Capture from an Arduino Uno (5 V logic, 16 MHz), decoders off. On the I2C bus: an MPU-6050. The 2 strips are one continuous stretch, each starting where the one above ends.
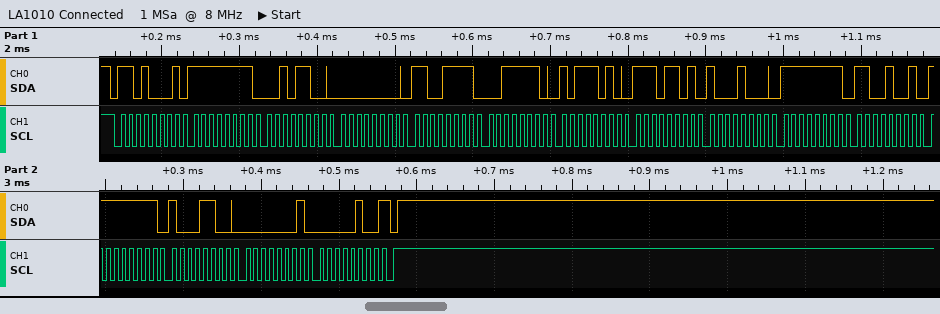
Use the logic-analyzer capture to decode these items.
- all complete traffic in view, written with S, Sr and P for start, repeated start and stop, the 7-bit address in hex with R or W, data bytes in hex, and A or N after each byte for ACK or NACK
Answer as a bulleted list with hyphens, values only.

- S 68R A FF A 2C A 00 A CF A 3E A BA A ED A 88 A FF A C9 A FF A 8C A 01 A 04 N P
